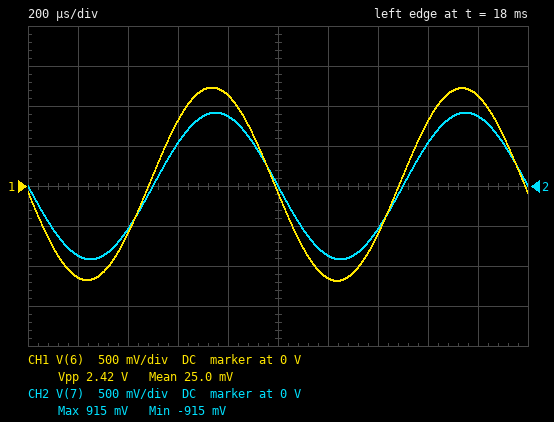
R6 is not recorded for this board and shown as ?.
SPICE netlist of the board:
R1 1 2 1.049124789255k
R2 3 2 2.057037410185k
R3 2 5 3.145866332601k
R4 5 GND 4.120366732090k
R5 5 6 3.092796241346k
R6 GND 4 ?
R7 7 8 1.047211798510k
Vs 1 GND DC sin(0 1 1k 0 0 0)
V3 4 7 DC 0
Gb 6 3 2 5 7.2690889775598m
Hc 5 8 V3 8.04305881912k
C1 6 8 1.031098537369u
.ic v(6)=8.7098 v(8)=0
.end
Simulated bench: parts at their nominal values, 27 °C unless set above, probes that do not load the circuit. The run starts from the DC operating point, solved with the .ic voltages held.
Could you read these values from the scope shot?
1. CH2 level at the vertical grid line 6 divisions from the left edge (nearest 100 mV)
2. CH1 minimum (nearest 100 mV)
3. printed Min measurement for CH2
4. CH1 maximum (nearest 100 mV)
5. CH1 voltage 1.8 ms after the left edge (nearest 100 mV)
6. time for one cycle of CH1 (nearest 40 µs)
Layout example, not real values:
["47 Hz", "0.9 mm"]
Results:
["-900 mV", "-1.2 V", "-915 mV", "1.2 V", "1.1 V", "1.00 ms"]
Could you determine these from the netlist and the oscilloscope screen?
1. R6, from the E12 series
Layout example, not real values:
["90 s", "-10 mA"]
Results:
["3.3 kΩ"]
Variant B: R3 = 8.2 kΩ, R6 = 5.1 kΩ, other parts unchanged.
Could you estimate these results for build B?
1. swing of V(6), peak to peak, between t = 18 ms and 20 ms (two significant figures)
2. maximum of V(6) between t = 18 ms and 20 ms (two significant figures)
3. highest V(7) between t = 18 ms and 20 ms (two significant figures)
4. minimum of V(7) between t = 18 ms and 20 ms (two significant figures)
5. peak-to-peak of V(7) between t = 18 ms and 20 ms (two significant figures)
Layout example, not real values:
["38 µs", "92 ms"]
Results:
["8.7 V", "4.4 V", "3.6 V", "-3.6 V", "7.3 V"]
